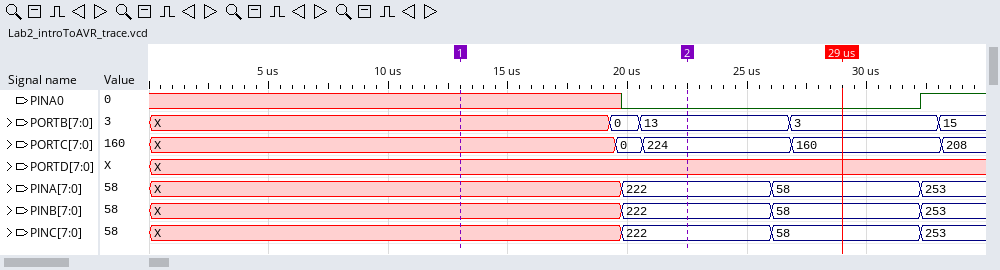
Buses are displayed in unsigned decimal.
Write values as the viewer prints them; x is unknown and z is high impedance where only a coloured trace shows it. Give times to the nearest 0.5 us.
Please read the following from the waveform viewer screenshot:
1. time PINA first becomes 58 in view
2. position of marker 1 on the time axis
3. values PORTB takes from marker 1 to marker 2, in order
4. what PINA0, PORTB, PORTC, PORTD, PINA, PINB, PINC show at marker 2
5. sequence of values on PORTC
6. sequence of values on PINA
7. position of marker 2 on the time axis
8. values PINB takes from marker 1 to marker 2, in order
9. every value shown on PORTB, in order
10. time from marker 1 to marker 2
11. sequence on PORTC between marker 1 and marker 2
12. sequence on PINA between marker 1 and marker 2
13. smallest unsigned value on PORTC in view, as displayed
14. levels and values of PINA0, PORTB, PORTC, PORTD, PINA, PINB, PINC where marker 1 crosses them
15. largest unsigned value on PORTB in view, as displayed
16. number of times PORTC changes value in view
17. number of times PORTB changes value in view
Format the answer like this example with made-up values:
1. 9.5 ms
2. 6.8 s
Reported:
1. 26 us
2. 13 us
3. X, 0, 13
4. PINA0=0, PORTB=13, PORTC=224, PORTD=X, PINA=222, PINB=222, PINC=222
5. X, 0, 224, 160, 208
6. X, 222, 58, 253
7. 22.5 us
8. X, 222
9. X, 0, 13, 3, 15
10. 9.5 us
11. X, 0, 224
12. X, 222
13. 0
14. PINA0=x, PORTB=X, PORTC=X, PORTD=X, PINA=X, PINB=X, PINC=X
15. 15
16. 4
17. 4
